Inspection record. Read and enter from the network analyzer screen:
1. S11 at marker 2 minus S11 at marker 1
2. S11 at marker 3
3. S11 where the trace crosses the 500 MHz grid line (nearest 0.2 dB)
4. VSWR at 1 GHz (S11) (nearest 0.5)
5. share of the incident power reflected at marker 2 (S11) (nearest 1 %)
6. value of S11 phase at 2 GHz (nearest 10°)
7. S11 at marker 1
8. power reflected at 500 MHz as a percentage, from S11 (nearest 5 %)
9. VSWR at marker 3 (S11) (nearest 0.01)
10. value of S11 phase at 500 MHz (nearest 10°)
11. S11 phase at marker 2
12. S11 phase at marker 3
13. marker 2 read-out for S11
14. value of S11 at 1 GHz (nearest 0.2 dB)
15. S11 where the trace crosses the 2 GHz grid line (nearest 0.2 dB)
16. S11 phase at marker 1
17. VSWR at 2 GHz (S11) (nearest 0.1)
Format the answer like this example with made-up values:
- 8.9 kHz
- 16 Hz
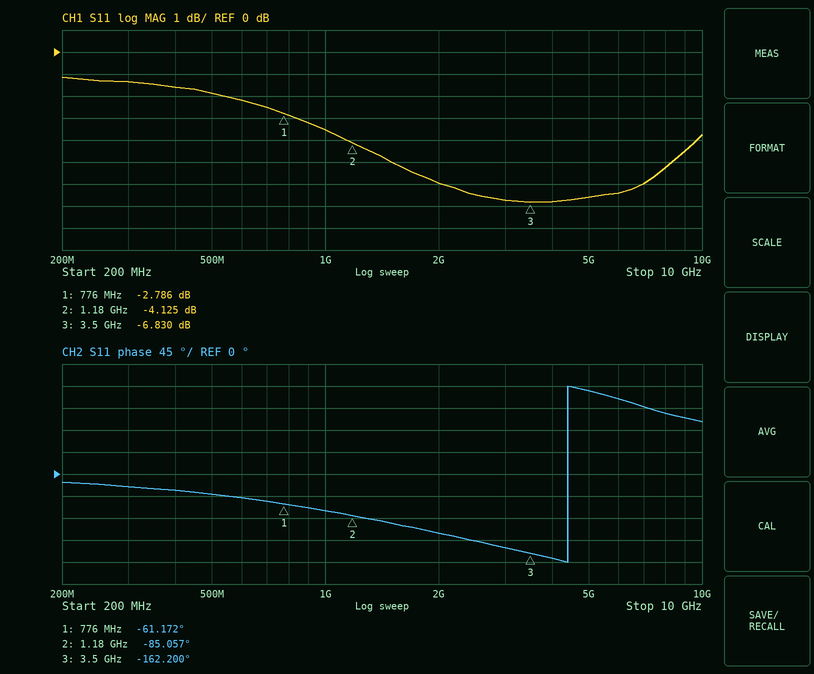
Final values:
- -1.339 dB
- -6.830 dB
- -1.8 dB
- 5.0
- 39 %
- -120°
- -2.786 dB
- 65 %
- 2.67
- -40°
- -85.057°
- -162.200°
- -4.125 dB
- -3.6 dB
- -6.0 dB
- -61.172°
- 3.0
